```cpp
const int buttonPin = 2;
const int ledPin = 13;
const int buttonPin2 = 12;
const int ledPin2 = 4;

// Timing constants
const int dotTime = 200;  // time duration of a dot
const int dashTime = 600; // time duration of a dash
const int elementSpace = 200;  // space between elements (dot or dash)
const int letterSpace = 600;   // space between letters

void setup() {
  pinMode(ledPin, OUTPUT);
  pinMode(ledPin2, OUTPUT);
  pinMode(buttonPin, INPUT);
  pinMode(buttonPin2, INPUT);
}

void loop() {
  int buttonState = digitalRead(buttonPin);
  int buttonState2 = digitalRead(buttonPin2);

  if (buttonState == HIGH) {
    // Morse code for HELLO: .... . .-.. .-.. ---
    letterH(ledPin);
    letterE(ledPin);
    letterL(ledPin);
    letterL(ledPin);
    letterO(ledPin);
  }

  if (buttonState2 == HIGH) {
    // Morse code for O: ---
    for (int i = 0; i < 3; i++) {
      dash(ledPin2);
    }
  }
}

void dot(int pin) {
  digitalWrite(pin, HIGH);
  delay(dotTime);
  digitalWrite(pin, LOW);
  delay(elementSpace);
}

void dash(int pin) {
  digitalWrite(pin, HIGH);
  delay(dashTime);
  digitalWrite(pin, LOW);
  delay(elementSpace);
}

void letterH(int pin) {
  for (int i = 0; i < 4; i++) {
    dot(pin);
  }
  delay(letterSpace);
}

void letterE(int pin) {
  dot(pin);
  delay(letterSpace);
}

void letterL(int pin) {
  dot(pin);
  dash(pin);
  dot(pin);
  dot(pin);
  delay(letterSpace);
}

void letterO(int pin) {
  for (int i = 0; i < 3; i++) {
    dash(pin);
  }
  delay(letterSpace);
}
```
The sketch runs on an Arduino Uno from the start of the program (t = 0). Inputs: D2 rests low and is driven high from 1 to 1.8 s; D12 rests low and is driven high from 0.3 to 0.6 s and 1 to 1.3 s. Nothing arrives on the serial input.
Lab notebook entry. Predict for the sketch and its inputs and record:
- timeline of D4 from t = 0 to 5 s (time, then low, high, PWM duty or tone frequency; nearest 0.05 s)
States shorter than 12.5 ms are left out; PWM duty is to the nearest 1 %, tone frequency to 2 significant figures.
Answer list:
0 s low; 0.3 s high; 0.9 s low; 1.1 s high; 1.7 s low; 1.9 s high; 2.5 s low
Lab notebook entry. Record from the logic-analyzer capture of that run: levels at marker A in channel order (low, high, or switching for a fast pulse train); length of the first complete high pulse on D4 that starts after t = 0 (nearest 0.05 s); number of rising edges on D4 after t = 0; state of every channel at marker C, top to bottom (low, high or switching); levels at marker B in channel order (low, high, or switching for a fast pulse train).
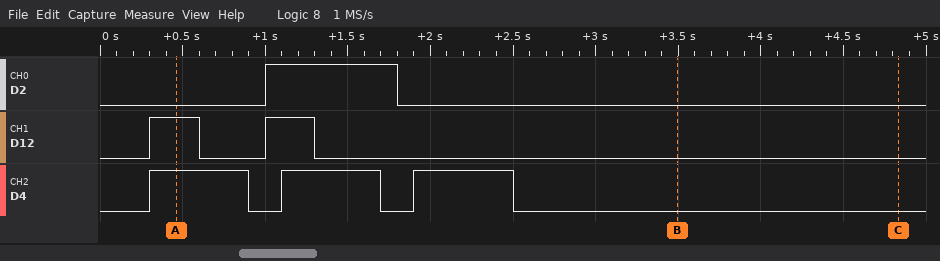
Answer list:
D2 low, D12 high, D4 high
0.60 s
3
D2 low, D12 low, D4 low
D2 low, D12 low, D4 low
